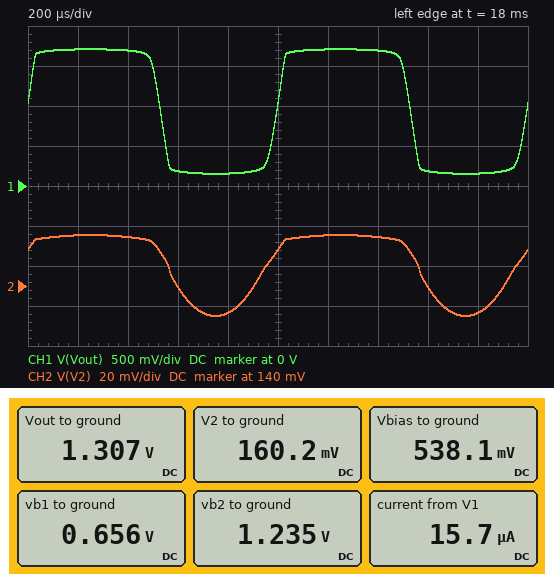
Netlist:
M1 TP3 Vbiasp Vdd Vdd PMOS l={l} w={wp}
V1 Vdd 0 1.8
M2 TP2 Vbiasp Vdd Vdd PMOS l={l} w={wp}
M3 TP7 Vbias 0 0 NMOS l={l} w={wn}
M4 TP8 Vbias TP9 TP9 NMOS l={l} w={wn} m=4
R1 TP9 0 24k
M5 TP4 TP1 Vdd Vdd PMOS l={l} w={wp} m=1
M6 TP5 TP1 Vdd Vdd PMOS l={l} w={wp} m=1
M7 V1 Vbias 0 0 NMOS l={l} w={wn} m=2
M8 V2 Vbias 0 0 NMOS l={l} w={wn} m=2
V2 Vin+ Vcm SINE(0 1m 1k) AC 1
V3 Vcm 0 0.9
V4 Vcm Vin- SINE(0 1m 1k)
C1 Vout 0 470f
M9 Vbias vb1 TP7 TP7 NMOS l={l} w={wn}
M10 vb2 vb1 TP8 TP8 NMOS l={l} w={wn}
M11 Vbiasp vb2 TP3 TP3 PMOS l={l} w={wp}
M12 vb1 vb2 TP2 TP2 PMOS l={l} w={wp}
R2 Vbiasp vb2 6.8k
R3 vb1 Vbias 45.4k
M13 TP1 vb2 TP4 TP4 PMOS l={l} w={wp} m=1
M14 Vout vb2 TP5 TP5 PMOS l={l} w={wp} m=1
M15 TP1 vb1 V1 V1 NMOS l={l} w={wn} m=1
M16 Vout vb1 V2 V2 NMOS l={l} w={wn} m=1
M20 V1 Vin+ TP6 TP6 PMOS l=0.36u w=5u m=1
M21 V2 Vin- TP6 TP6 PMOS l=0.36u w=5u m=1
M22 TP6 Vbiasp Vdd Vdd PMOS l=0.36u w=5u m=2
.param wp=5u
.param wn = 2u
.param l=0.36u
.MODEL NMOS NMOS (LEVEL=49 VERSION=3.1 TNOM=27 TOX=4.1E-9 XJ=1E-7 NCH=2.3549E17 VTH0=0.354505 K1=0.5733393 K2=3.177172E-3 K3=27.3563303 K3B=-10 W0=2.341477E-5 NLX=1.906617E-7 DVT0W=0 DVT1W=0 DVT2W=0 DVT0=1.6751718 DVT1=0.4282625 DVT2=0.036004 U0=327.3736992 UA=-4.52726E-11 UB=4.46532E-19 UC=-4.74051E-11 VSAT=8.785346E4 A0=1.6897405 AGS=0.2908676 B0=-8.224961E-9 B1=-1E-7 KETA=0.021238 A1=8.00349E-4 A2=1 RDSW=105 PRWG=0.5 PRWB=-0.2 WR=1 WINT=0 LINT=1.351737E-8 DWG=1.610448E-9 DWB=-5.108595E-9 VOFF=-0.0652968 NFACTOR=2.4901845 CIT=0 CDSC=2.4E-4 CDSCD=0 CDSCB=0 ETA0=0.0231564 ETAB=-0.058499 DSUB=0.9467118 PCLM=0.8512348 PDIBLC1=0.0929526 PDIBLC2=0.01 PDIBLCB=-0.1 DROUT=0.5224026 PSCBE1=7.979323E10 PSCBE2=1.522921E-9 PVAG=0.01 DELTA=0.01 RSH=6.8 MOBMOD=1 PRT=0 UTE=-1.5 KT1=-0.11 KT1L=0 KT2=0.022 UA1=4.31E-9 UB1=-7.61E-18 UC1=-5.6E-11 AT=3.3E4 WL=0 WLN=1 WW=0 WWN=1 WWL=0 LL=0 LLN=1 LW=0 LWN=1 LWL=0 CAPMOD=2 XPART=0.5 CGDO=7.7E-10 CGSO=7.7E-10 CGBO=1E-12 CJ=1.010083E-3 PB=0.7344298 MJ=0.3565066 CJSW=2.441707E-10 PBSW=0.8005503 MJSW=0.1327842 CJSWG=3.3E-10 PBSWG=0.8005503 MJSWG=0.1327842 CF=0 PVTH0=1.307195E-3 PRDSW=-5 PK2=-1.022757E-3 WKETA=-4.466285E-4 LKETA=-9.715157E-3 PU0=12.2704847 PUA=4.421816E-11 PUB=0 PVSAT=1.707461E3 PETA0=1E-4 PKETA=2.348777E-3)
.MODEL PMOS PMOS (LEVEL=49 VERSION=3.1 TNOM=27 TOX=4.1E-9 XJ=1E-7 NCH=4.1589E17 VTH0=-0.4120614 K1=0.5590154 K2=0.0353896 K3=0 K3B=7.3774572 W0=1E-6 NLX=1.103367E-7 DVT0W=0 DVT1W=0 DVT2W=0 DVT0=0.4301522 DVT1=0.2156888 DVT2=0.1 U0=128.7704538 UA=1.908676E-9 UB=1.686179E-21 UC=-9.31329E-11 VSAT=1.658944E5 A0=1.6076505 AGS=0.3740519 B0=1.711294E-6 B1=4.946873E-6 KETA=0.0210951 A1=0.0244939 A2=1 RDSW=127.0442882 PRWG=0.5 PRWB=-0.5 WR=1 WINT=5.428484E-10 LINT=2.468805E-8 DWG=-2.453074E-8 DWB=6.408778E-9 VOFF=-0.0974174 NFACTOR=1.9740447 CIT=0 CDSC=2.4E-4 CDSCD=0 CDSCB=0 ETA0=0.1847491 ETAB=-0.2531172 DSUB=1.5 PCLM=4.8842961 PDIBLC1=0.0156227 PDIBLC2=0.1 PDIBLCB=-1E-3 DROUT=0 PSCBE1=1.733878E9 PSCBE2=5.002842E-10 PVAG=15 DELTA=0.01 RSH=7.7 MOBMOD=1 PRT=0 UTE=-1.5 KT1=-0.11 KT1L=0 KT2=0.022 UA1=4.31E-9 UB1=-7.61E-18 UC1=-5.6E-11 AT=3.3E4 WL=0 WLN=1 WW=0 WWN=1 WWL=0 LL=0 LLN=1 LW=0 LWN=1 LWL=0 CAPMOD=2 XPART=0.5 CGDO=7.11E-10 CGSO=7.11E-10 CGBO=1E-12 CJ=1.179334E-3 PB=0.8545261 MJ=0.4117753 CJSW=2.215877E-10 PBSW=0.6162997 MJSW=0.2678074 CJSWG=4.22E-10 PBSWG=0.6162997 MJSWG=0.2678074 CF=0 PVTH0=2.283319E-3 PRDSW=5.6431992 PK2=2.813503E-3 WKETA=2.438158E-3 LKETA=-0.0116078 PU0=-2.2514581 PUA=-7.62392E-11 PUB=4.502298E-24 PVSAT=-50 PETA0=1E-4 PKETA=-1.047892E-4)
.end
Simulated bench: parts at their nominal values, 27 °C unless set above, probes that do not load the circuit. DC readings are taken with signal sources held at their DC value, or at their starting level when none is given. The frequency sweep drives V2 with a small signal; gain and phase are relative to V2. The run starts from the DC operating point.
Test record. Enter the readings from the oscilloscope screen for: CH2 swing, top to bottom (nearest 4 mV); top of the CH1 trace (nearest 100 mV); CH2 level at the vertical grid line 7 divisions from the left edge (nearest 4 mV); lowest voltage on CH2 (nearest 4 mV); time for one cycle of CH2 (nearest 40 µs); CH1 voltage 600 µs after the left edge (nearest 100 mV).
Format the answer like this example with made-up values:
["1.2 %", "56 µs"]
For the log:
["40 mV", "1.7 V", "164 mV", "124 mV", "1.00 ms", "200 mV"]
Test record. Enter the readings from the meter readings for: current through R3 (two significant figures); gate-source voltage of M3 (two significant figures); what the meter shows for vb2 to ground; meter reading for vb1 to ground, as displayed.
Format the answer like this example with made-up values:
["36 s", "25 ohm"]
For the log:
["2.6 µA", "540 mV", "1.235 V", "0.656 V"]
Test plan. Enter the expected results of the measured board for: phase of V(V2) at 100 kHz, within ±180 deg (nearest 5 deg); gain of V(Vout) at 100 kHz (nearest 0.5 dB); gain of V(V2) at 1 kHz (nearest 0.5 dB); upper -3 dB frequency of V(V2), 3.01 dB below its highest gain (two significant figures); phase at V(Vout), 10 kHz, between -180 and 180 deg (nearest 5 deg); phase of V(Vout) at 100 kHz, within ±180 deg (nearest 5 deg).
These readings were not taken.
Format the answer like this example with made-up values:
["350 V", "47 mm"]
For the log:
["-55 deg", "46.5 dB", "23.0 dB", "12 kHz", "-40 deg", "-85 deg"]
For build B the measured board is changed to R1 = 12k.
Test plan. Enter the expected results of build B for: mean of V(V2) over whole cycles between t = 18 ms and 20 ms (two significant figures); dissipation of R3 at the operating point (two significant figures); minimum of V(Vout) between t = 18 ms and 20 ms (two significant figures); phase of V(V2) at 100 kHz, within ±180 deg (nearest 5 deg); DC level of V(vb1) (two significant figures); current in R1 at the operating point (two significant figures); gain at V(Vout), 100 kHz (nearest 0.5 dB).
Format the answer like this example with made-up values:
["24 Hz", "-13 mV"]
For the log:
["280 mV", "1.5 µW", "270 mV", "-65 deg", "830 mV", "5.6 µA", "51.0 dB"]
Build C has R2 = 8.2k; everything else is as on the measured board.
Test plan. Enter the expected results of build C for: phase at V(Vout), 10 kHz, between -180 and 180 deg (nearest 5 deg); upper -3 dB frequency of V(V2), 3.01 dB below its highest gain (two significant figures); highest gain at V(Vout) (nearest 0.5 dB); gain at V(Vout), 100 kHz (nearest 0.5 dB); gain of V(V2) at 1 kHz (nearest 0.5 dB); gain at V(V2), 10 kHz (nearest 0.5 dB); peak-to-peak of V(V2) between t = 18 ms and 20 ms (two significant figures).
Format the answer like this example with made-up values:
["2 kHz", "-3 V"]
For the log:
["-35 deg", "14 kHz", "63.5 dB", "46.0 dB", "22.0 dB", "20.0 dB", "38 mV"]
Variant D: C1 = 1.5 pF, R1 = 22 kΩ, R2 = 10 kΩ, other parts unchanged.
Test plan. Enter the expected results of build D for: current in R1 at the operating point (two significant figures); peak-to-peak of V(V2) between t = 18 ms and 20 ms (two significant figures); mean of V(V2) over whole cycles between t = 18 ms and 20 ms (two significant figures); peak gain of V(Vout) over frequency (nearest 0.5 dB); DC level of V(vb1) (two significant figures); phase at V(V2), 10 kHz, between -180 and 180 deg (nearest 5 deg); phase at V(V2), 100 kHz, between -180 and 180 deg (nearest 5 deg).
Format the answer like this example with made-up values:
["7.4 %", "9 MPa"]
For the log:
["2.8 µA", "37 mV", "160 mV", "62.5 dB", "670 mV", "-55 deg", "-30 deg"]
